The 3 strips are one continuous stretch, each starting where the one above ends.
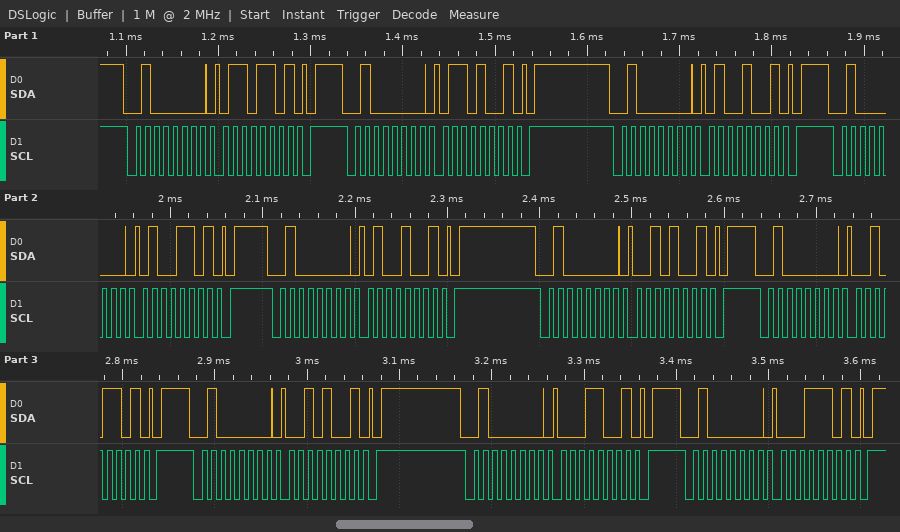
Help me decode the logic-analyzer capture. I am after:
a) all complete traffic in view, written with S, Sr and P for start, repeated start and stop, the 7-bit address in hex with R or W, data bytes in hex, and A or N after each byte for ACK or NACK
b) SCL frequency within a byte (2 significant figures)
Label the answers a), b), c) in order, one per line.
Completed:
a) S 20W A 6D A P S 20W A 69 A P S 20W A 49 A P S 20W A 4D A P S 20W A 49 A P S 20W A 29 A P S 20W A 2D A P S 20W A 29 A P S 20W A 19 A P S 20W A 1D A P
b) 100 kHz
